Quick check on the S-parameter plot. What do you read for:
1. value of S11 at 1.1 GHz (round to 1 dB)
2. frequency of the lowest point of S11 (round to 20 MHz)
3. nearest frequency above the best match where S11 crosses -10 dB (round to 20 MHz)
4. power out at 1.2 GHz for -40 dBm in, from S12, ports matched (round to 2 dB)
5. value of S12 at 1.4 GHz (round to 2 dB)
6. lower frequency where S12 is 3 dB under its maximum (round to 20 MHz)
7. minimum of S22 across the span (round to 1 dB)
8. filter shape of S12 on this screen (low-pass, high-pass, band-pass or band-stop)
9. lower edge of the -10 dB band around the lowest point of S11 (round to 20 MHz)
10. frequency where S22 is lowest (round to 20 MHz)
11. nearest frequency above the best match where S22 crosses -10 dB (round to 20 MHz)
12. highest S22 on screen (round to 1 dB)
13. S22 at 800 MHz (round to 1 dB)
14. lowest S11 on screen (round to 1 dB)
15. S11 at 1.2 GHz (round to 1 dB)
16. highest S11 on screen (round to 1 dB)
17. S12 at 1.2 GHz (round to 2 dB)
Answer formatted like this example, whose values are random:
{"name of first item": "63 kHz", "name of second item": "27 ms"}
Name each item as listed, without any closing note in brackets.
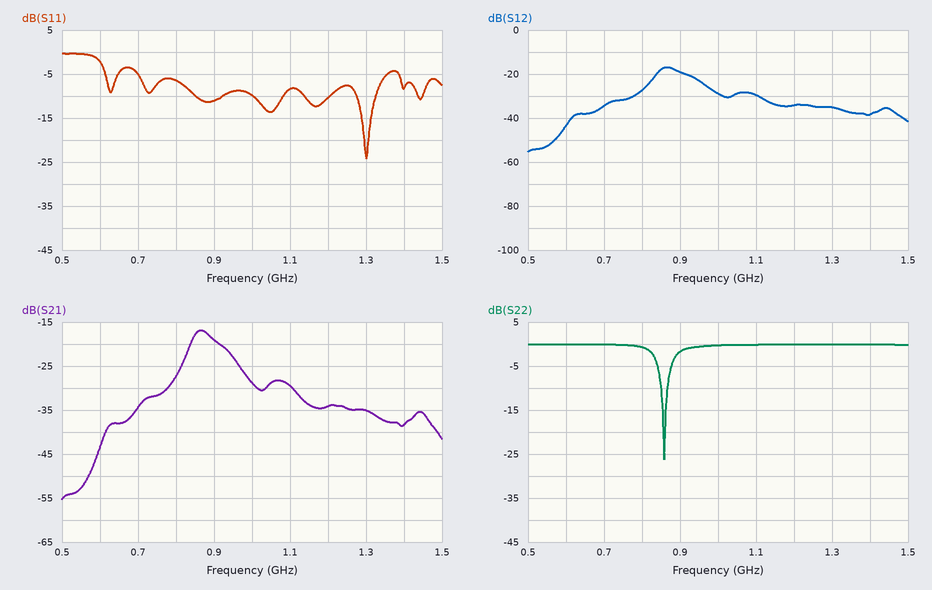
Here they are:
{"value of S11 at 1.1 GHz": "-8 dB", "frequency of the lowest point of S11": "1.30 GHz", "nearest frequency above the best match where S11 crosses -10 dB": "1.32 GHz", "power out at 1.2 GHz for -40 dBm in, from S12, ports matched": "-74 dBm", "value of S12 at 1.4 GHz": "-38 dB", "lower frequency where S12 is 3 dB under its maximum": "840 MHz", "minimum of S22 across the span": "-26 dB", "filter shape of S12 on this screen": "band-pass", "lower edge of the -10 dB band around the lowest point of S11": "1.28 GHz", "frequency where S22 is lowest": "860 MHz", "nearest frequency above the best match where S22 crosses -10 dB": "860 MHz", "highest S22 on screen": "0 dB", "S22 at 800 MHz": "-1 dB", "lowest S11 on screen": "-24 dB", "S11 at 1.2 GHz": "-10 dB", "highest S11 on screen": "0 dB", "S12 at 1.2 GHz": "-34 dB"}
